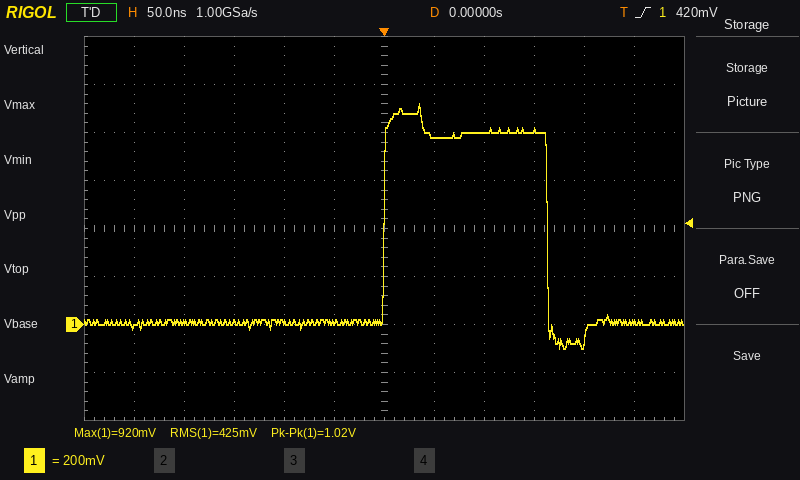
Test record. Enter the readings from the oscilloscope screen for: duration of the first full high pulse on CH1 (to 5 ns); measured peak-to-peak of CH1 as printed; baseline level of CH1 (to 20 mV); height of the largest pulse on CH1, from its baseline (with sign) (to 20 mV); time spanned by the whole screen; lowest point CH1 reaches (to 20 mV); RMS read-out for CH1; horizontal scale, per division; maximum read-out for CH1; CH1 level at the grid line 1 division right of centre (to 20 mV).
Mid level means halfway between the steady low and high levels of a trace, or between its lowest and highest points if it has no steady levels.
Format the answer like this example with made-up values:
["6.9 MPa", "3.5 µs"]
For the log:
["165 ns", "1.02 V", "0 mV", "+920 mV", "600 ns", "-100 mV", "425 mV", "50 ns", "920 mV", "780 mV"]
